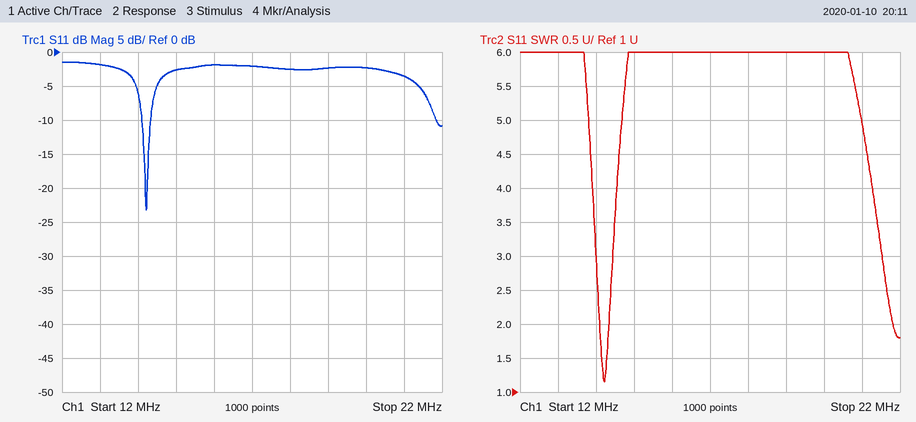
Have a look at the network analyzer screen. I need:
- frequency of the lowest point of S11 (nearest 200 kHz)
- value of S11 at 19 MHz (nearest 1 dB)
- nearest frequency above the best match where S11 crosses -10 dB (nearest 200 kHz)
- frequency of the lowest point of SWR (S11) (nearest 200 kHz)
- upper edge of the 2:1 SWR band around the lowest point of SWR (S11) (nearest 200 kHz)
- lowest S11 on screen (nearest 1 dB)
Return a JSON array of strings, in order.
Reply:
["14.2 MHz", "-2 dB", "14.4 MHz", "14.2 MHz", "14.4 MHz", "-23 dB"]
